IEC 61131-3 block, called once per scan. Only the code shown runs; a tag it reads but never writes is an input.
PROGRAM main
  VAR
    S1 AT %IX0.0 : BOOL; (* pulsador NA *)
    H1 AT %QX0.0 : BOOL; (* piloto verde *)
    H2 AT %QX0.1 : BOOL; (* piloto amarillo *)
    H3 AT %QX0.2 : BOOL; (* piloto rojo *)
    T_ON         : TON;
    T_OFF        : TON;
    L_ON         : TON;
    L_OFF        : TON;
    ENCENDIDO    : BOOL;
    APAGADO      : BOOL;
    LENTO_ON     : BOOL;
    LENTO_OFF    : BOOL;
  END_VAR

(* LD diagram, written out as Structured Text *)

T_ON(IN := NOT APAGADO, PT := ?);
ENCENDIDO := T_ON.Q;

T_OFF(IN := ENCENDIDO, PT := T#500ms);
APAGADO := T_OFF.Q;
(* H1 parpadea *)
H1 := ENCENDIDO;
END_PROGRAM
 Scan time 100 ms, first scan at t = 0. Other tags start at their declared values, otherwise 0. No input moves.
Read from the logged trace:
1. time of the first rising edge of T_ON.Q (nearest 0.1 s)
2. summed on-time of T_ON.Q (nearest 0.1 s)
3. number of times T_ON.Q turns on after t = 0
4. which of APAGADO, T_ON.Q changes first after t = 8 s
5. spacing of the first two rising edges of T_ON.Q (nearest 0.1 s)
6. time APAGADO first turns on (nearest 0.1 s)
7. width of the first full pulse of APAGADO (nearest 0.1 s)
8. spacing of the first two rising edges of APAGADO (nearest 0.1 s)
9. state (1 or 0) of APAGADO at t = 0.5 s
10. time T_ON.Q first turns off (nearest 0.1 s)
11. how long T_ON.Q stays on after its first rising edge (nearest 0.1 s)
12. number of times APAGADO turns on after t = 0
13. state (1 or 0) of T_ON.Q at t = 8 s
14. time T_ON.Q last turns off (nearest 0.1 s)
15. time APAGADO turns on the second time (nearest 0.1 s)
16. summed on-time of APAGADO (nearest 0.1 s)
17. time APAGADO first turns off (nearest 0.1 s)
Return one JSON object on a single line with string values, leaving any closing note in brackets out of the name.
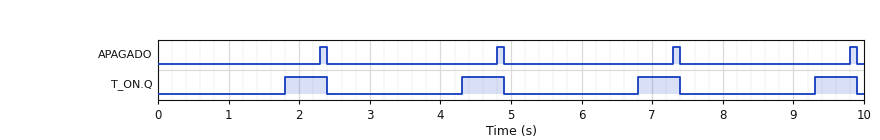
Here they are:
{"time of the first rising edge of T_ON.Q": "1.8 s", "summed on-time of T_ON.Q": "2.4 s", "number of times T_ON.Q turns on after t = 0": "4", "which of APAGADO, T_ON.Q changes first after t = 8 s": "T_ON.Q", "spacing of the first two rising edges of T_ON.Q": "2.5 s", "time APAGADO first turns on": "2.3 s", "width of the first full pulse of APAGADO": "0.1 s", "spacing of the first two rising edges of APAGADO": "2.5 s", "state (1 or 0) of APAGADO at t = 0.5 s": "0", "time T_ON.Q first turns off": "2.4 s", "how long T_ON.Q stays on after its first rising edge": "0.6 s", "number of times APAGADO turns on after t = 0": "4", "state (1 or 0) of T_ON.Q at t = 8 s": "0", "time T_ON.Q last turns off": "9.9 s", "time APAGADO turns on the second time": "4.8 s", "summed on-time of APAGADO": "0.4 s", "time APAGADO first turns off": "2.4 s"}
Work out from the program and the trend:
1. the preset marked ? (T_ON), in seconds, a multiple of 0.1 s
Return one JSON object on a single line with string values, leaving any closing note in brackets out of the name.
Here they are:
{"the preset marked ? (T_ON), in seconds, a multiple of 0.1 s": "1.8 s"}
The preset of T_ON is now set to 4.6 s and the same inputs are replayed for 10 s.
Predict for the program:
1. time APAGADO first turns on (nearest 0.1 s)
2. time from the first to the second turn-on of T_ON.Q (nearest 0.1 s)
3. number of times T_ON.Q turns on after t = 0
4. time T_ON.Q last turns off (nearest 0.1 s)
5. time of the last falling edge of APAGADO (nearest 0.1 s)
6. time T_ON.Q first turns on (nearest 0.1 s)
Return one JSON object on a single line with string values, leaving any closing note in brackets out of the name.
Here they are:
{"time APAGADO first turns on": "5.1 s", "time from the first to the second turn-on of T_ON.Q": "5.3 s", "number of times T_ON.Q turns on after t = 0": "2", "time T_ON.Q last turns off": "5.2 s", "time of the last falling edge of APAGADO": "5.2 s", "time T_ON.Q first turns on": "4.6 s"}
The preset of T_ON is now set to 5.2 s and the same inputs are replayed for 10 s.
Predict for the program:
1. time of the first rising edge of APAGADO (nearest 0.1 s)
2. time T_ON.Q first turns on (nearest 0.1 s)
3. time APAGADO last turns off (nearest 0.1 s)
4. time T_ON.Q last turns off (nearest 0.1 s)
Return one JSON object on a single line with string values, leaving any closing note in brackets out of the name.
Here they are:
{"time of the first rising edge of APAGADO": "5.7 s", "time T_ON.Q first turns on": "5.2 s", "time APAGADO last turns off": "5.8 s", "time T_ON.Q last turns off": "5.8 s"}
